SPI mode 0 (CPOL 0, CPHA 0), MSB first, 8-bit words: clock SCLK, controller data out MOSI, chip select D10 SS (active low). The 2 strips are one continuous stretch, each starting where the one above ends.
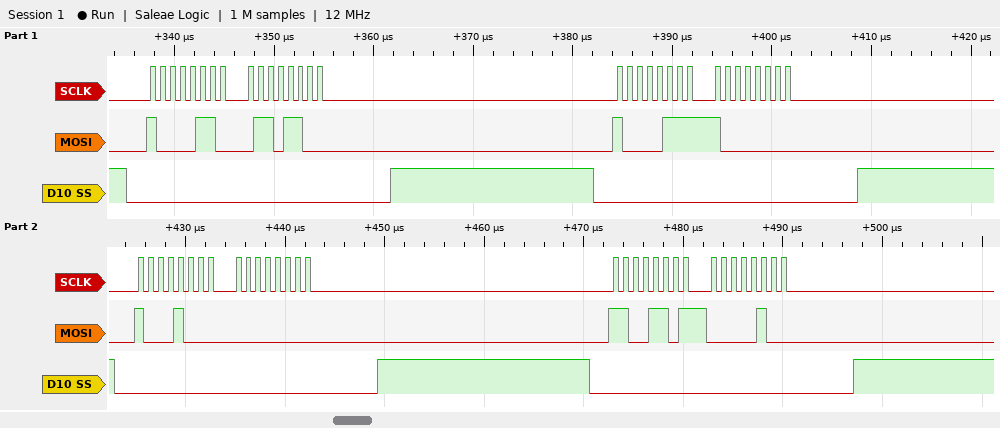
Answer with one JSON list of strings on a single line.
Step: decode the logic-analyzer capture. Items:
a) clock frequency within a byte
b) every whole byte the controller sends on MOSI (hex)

["1 MHz", "86 6C 87 80 88 00 CD 04"]
